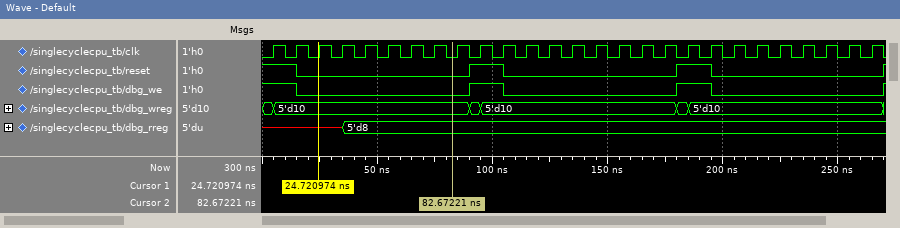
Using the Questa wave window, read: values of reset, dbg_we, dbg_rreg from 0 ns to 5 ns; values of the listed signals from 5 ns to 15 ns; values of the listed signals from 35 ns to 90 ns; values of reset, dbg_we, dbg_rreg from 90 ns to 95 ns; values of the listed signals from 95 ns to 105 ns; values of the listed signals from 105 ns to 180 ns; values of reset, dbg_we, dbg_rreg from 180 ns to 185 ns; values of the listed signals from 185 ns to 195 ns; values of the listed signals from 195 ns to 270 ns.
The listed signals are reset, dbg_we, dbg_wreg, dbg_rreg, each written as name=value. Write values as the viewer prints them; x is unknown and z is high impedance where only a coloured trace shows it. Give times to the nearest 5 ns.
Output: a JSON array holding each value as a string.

["reset=1, dbg_we=1, dbg_rreg=x", "reset=1, dbg_we=1, dbg_wreg=5'd10, dbg_rreg=x", "reset=0, dbg_we=0, dbg_wreg=5'd10, dbg_rreg=5'd8", "reset=1, dbg_we=1, dbg_rreg=5'd8", "reset=1, dbg_we=1, dbg_wreg=5'd10, dbg_rreg=5'd8", "reset=0, dbg_we=0, dbg_wreg=5'd10, dbg_rreg=5'd8", "reset=1, dbg_we=1, dbg_rreg=5'd8", "reset=1, dbg_we=1, dbg_wreg=5'd10, dbg_rreg=5'd8", "reset=0, dbg_we=0, dbg_wreg=5'd10, dbg_rreg=5'd8"]
